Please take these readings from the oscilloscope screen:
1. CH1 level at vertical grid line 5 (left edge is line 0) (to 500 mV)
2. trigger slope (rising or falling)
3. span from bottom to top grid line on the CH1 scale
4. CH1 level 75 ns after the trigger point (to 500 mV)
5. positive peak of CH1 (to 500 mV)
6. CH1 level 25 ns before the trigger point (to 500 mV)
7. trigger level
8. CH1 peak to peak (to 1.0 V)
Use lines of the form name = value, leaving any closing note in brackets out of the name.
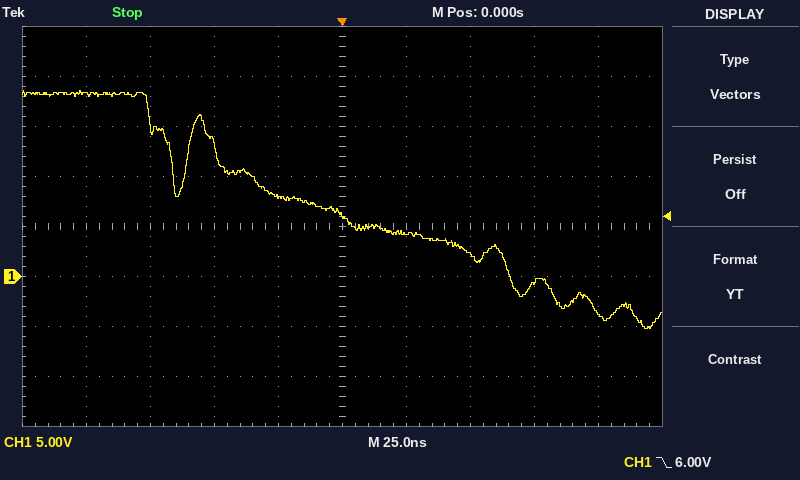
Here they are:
CH1 level at vertical grid line 5 (left edge is line 0) = 6.0 V
trigger slope = falling
span from bottom to top grid line on the CH1 scale = 40 V
CH1 level 75 ns after the trigger point = -500 mV
positive peak of CH1 = 18.5 V
CH1 level 25 ns before the trigger point = 8.0 V
trigger level = 6.00 V
CH1 peak to peak = 24.0 V
